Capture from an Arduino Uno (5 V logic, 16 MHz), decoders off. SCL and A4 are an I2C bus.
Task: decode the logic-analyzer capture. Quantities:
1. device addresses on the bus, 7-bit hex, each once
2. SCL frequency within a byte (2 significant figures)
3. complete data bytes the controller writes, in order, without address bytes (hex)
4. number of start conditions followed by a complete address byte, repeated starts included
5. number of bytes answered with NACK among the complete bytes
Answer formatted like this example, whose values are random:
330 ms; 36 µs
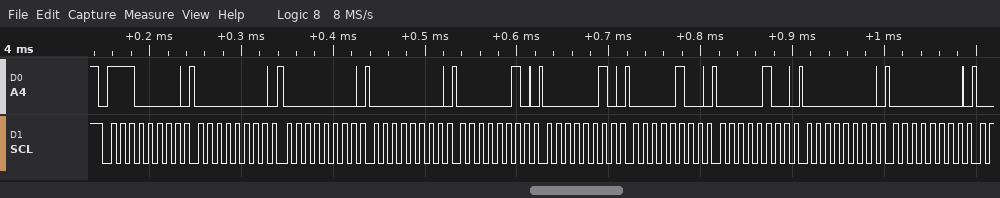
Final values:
0x70; 100 kHz; 00 00 00 02 02 04 04 00 00; 1; 0
